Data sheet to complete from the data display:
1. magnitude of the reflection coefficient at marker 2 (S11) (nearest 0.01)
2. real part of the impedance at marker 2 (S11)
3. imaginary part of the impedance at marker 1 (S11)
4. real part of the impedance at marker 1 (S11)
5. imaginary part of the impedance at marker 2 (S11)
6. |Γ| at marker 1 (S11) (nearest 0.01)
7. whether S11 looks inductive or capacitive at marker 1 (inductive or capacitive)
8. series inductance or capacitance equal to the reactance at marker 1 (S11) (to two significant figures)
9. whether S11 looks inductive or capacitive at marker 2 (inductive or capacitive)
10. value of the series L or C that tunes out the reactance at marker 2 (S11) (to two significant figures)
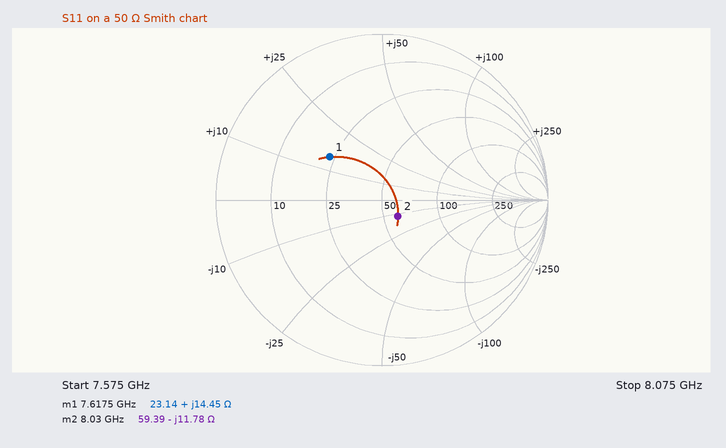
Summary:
0.14
59.39 Ω
+14.45 Ω
23.14 Ω
-11.78 Ω
0.41
inductive
300 pH
capacitive
230 pH
